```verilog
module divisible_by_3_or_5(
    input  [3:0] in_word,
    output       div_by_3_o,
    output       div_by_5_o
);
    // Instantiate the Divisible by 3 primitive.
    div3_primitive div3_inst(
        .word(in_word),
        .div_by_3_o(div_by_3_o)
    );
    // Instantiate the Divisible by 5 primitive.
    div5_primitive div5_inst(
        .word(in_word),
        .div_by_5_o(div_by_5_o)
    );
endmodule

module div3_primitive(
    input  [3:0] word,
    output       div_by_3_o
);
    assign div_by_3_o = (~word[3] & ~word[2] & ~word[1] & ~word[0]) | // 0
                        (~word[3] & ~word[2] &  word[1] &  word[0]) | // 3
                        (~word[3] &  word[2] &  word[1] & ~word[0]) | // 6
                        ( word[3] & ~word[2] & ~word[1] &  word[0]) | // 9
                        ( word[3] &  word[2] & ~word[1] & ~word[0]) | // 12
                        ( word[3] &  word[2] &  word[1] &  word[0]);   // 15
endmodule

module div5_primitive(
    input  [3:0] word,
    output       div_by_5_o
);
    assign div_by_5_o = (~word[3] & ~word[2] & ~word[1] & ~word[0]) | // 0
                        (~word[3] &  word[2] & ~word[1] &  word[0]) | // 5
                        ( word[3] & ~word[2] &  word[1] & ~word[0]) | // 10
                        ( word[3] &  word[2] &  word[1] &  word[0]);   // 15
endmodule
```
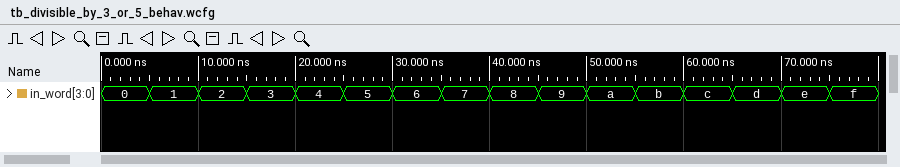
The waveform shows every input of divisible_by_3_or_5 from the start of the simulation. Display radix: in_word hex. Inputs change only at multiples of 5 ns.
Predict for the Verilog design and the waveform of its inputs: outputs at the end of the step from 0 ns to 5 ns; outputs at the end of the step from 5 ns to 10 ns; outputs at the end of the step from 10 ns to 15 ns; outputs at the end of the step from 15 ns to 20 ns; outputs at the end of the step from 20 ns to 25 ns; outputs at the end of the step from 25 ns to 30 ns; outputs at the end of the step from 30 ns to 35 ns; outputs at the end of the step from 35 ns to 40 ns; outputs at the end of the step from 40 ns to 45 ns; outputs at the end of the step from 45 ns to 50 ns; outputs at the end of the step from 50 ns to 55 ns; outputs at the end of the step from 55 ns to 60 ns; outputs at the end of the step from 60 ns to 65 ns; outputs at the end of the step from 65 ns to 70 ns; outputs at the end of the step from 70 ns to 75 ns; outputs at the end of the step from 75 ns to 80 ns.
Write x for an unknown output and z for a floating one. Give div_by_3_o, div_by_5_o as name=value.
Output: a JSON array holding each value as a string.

["div_by_3_o=1, div_by_5_o=1", "div_by_3_o=0, div_by_5_o=0", "div_by_3_o=0, div_by_5_o=0", "div_by_3_o=1, div_by_5_o=0", "div_by_3_o=0, div_by_5_o=0", "div_by_3_o=0, div_by_5_o=1", "div_by_3_o=1, div_by_5_o=0", "div_by_3_o=0, div_by_5_o=0", "div_by_3_o=0, div_by_5_o=0", "div_by_3_o=1, div_by_5_o=0", "div_by_3_o=0, div_by_5_o=1", "div_by_3_o=0, div_by_5_o=0", "div_by_3_o=1, div_by_5_o=0", "div_by_3_o=0, div_by_5_o=0", "div_by_3_o=0, div_by_5_o=0", "div_by_3_o=1, div_by_5_o=1"]
